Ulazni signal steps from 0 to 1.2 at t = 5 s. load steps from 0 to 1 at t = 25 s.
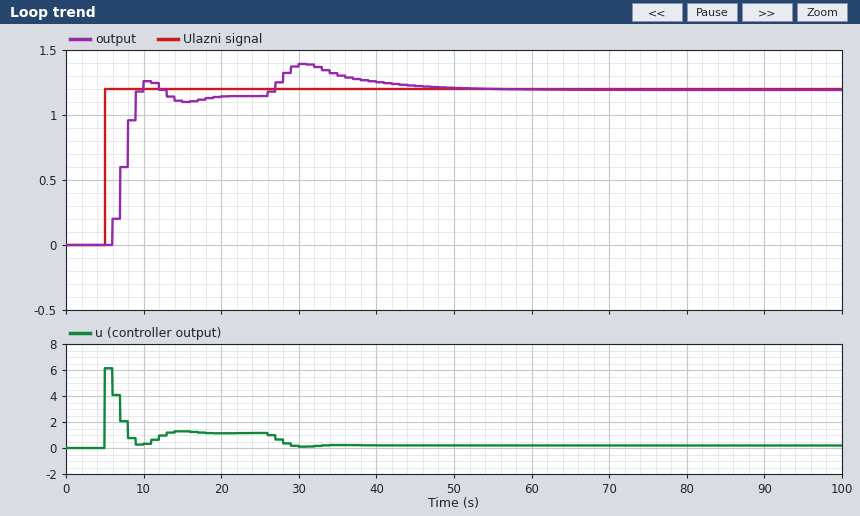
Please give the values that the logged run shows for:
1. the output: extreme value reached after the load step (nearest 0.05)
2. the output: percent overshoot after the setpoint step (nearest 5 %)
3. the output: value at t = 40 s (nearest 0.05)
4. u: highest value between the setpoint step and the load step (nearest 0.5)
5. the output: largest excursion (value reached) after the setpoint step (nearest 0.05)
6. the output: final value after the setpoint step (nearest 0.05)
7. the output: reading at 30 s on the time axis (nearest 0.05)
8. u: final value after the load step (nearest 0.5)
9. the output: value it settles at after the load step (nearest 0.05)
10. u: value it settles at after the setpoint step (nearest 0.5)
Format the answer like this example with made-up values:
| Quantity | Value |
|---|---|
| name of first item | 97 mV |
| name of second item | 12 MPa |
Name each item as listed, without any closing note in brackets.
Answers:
| Quantity | Value |
|---|---|
| the output: extreme value reached after the load step | 1.40 |
| the output: percent overshoot after the setpoint step | 10 % |
| the output: value at t = 40 s | 1.25 |
| u: highest value between the setpoint step and the load step | 6.0 |
| the output: largest excursion (value reached) after the setpoint step | 1.25 |
| the output: final value after the setpoint step | 1.15 |
| the output: reading at 30 s on the time axis | 1.40 |
| u: final value after the load step | 0.0 |
| the output: value it settles at after the load step | 1.20 |
| u: value it settles at after the setpoint step | 1.0 |
